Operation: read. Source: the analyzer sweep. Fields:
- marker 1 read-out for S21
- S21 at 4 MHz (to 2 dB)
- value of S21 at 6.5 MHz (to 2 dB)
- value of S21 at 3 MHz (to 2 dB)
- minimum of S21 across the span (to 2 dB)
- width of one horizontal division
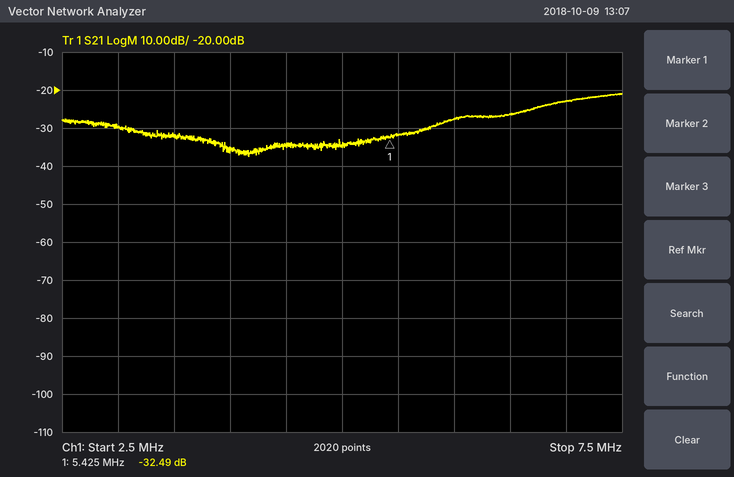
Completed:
-32.49 dB
-36 dB
-26 dB
-30 dB
-38 dB
500 kHz
